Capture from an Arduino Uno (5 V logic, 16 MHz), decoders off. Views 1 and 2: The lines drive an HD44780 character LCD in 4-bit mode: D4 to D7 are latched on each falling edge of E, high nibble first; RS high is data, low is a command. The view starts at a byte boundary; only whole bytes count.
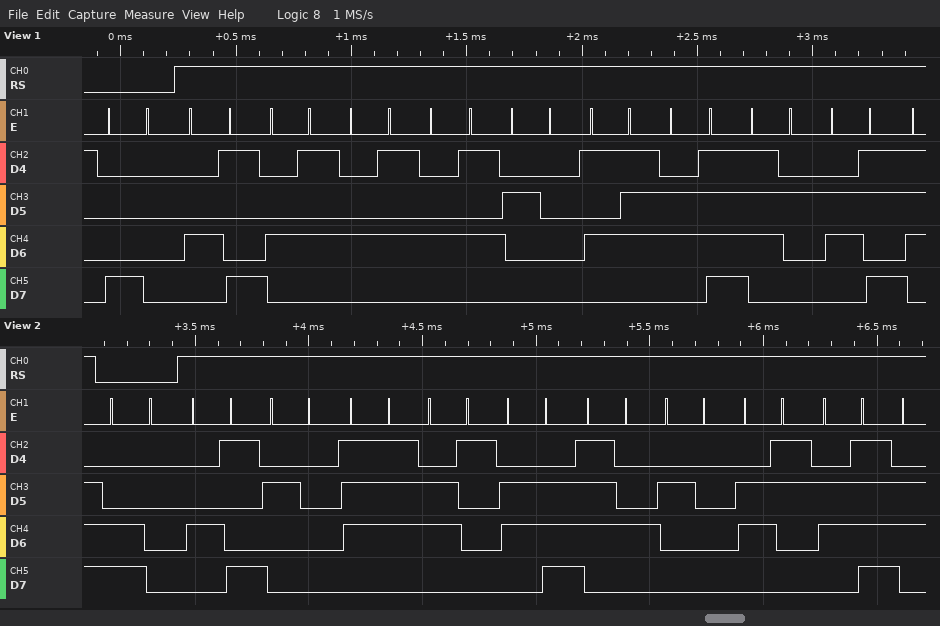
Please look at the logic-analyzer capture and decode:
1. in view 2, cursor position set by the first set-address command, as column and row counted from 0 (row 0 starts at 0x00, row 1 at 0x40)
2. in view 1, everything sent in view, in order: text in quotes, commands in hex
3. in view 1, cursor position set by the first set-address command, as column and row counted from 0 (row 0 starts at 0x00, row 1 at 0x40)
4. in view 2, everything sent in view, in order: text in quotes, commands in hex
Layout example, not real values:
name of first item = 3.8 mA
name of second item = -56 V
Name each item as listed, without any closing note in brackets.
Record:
in view 2, cursor position set by the first set-address command, as column and row counted from 0 = column 0, row 1
in view 1, everything sent in view, in order: text in quotes, commands in hex = 0x80 "IEEE Work"
in view 1, cursor position set by the first set-address command, as column and row counted from 0 = column 0, row 0
in view 2, everything sent in view, in order: text in quotes, commands in hex = 0xC0 "I want co"
